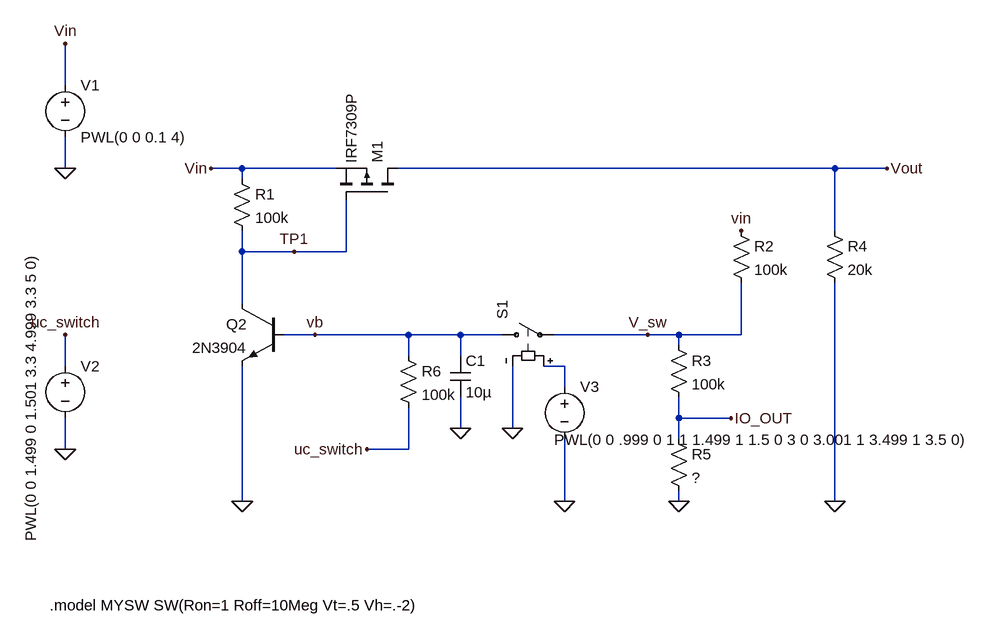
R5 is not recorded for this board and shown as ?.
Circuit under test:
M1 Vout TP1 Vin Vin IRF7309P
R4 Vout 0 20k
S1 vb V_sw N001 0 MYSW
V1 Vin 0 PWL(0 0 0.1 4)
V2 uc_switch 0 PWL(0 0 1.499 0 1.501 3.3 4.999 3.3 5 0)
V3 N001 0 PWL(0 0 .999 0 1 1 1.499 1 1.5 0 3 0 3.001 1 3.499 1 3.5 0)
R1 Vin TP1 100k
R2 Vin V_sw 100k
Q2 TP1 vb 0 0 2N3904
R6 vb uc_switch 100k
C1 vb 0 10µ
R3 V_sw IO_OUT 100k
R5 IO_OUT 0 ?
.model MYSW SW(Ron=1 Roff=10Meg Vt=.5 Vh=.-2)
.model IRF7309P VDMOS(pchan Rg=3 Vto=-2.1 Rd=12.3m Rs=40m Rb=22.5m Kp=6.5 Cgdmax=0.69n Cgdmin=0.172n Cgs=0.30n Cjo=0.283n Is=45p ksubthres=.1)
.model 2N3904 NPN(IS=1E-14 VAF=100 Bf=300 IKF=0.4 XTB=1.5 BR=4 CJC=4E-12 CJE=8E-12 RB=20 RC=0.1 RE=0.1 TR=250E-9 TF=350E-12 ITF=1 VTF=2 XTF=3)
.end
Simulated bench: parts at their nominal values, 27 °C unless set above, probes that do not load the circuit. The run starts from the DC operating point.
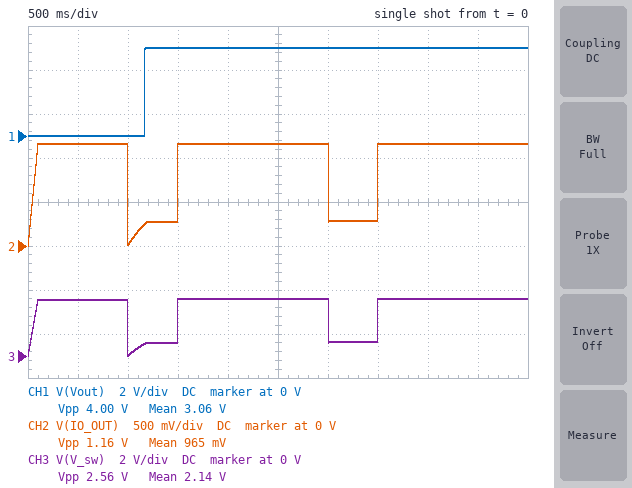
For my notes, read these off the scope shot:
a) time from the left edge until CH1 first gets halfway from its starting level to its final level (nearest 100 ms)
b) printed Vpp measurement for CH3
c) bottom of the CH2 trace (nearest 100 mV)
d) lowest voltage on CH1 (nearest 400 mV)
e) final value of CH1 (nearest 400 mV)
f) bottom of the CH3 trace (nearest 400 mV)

1.2 s
2.56 V
0 V
0 V
4.0 V
0 V
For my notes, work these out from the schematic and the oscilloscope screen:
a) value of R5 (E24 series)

82 kΩ
